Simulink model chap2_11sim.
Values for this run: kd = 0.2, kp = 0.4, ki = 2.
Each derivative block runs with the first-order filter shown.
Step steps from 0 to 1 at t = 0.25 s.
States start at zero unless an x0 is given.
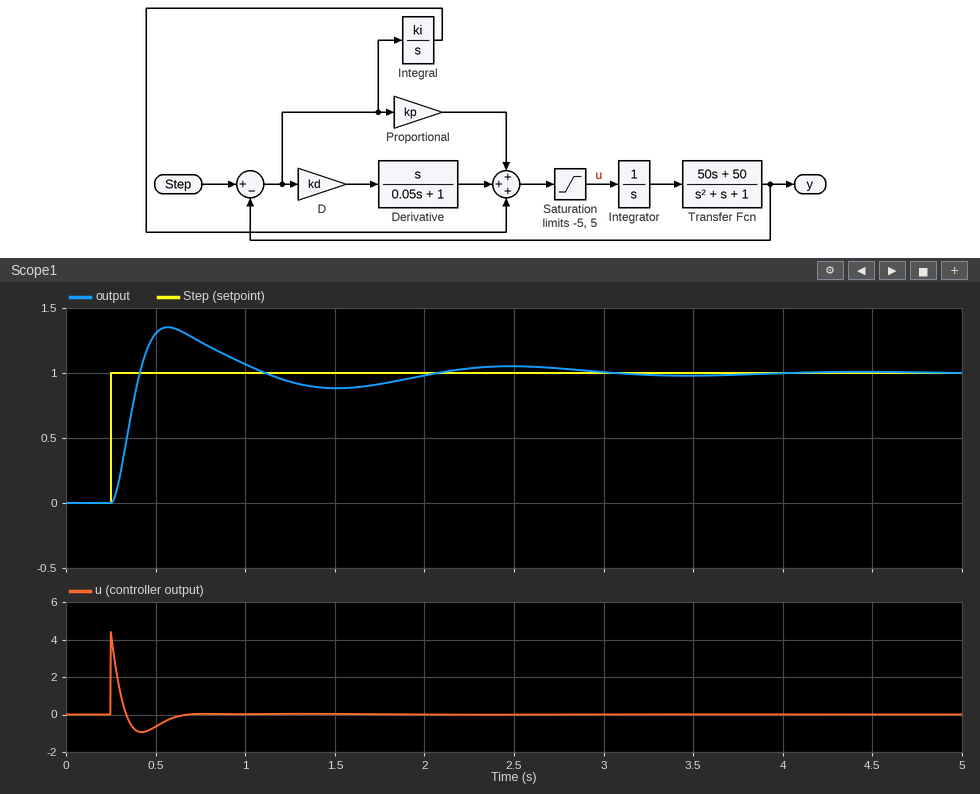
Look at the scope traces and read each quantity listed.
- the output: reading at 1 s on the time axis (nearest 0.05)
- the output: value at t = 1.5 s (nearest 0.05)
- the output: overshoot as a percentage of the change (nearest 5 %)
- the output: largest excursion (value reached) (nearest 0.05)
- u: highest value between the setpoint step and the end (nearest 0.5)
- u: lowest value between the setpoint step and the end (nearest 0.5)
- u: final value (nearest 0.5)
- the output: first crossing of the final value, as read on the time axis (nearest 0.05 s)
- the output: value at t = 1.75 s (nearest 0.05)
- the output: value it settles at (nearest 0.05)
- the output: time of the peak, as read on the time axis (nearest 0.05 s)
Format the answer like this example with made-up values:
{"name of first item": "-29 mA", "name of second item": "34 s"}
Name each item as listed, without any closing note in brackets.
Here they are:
{"the output: reading at 1 s on the time axis": "1.05", "the output: value at t = 1.5 s": "0.90", "the output: overshoot as a percentage of the change": "35 %", "the output: largest excursion (value reached)": "1.35", "u: highest value between the setpoint step and the end": "4.5", "u: lowest value between the setpoint step and the end": "-1.0", "u: final value": "0.0", "the output: first crossing of the final value, as read on the time axis": "0.40 s", "the output: value at t = 1.75 s": "0.90", "the output: value it settles at": "1.00", "the output: time of the peak, as read on the time axis": "0.55 s"}
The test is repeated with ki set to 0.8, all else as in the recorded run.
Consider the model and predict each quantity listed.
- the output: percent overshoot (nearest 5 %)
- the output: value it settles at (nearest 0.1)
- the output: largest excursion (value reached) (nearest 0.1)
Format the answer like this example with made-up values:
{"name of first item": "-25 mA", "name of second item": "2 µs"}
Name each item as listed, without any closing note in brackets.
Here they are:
{"the output: percent overshoot": "25 %", "the output: value it settles at": "1.0", "the output: largest excursion (value reached)": "1.3"}
